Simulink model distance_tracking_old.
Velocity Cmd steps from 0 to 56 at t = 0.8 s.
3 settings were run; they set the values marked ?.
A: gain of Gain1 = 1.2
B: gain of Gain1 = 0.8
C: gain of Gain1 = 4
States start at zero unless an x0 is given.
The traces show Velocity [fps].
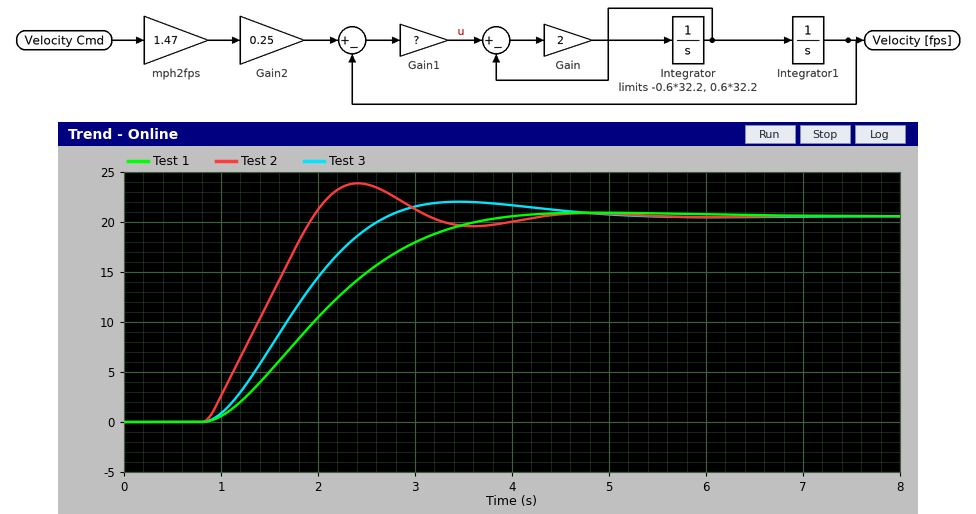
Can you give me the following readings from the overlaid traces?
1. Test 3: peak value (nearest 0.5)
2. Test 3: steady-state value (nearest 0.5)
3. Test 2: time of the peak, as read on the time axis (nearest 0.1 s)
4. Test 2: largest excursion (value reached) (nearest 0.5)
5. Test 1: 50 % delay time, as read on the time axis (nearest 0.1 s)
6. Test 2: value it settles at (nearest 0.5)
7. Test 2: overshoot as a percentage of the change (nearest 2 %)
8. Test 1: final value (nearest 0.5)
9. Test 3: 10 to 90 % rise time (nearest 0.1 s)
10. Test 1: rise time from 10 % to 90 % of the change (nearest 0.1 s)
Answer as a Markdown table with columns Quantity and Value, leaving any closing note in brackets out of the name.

| Quantity | Value |
|---|---|
| Test 3: peak value | 22.0 |
| Test 3: steady-state value | 20.5 |
| Test 2: time of the peak, as read on the time axis | 2.4 s |
| Test 2: largest excursion (value reached) | 24.0 |
| Test 1: 50 % delay time, as read on the time axis | 2.0 s |
| Test 2: value it settles at | 20.5 |
| Test 2: overshoot as a percentage of the change | 16 % |
| Test 1: final value | 20.5 |
| Test 3: 10 to 90 % rise time | 1.3 s |
| Test 1: rise time from 10 % to 90 % of the change | 1.9 s |
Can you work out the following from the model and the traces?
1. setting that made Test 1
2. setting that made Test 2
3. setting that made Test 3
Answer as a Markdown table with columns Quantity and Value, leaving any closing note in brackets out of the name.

| Quantity | Value |
|---|---|
| setting that made Test 1 | B |
| setting that made Test 2 | C |
| setting that made Test 3 | A |
